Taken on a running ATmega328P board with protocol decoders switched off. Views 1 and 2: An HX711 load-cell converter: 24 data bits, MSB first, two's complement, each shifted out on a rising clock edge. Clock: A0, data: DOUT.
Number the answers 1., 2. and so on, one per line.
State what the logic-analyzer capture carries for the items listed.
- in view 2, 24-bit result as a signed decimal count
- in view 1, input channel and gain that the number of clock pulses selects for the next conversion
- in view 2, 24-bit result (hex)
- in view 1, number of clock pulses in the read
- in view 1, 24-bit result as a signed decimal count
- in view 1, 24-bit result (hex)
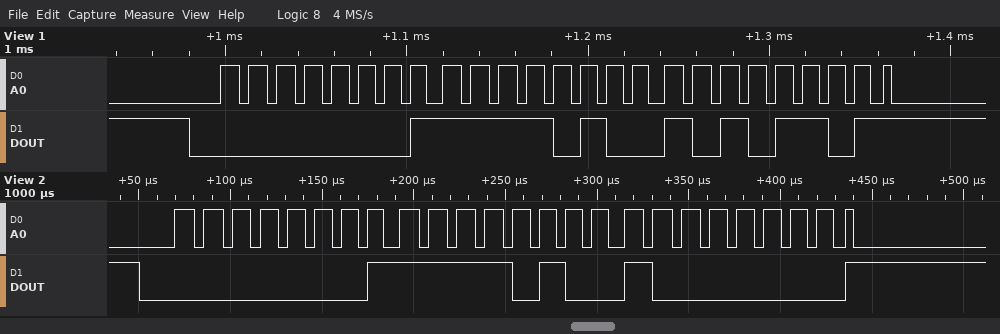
1. 128128
2. channel A, gain 128
3. 0x01F480
4. 25
5. 128173
6. 0x01F4AD
